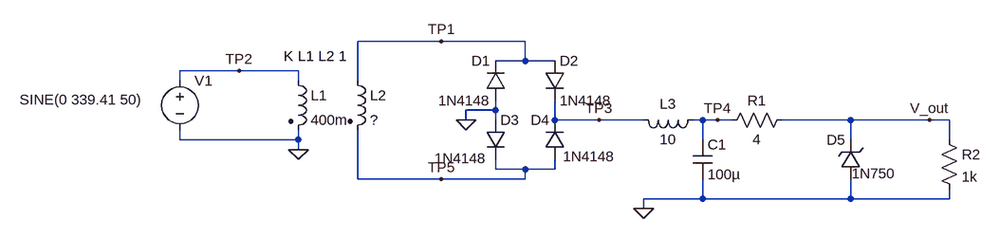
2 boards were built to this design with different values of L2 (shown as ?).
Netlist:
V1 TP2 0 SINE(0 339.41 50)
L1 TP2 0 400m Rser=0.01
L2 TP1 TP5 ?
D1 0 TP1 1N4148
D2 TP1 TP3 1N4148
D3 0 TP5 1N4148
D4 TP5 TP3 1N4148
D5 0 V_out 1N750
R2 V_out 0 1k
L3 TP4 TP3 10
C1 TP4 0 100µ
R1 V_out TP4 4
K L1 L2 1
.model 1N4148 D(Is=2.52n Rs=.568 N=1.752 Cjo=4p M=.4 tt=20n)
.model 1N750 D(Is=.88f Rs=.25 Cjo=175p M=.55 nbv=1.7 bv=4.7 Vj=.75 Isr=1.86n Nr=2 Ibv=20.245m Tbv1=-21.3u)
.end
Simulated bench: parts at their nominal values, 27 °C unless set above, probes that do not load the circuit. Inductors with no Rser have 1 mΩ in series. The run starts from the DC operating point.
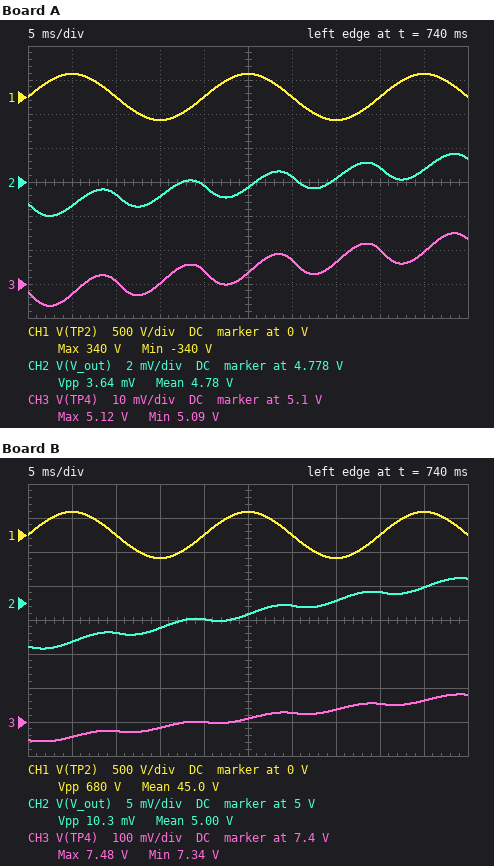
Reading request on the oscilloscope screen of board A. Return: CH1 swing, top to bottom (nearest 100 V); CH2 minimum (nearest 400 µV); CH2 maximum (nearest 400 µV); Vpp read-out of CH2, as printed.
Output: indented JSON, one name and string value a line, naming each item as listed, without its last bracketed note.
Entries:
{
  "CH1 swing, top to bottom": "700 V",
  "CH2 minimum": "4.7760 V",
  "CH2 maximum": "4.7796 V",
  "Vpp read-out of CH2, as printed": "3.64 mV"
}
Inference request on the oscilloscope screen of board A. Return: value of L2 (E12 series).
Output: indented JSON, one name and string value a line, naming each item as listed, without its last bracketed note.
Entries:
{
  "value of L2": "470 µH"
}
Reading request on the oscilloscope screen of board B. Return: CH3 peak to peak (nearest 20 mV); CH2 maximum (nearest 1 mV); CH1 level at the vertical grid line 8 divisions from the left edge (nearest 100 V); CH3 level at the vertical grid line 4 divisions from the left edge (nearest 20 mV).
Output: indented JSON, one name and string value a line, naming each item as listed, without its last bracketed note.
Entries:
{
  "CH3 peak to peak": "140 mV",
  "CH2 maximum": "5.004 V",
  "CH1 level at the vertical grid line 8 divisions from the left edge": "0 V",
  "CH3 level at the vertical grid line 4 divisions from the left edge": "7.40 V"
}
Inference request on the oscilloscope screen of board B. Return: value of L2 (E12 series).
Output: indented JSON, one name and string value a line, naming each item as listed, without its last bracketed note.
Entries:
{
  "value of L2": "2.2 mH"
}
